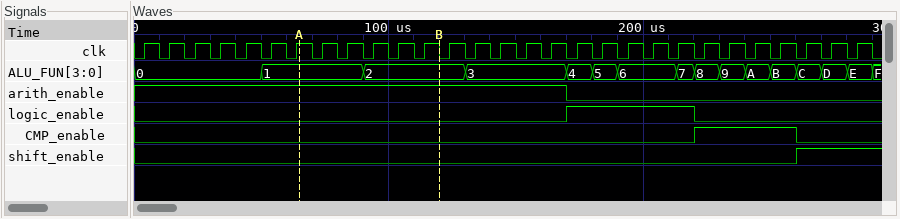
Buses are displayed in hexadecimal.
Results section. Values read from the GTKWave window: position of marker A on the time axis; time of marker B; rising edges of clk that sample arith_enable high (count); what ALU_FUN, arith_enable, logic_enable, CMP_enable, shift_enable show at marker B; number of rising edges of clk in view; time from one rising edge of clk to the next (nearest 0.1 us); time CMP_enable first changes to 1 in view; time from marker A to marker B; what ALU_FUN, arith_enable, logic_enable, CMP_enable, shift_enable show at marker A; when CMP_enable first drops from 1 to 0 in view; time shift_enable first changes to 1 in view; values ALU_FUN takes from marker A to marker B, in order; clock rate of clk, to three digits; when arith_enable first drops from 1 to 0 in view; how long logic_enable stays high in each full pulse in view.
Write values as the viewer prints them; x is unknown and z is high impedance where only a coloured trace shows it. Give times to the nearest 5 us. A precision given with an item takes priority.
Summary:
65 us
120 us
17
ALU_FUN=2, arith_enable=1, logic_enable=0, CMP_enable=0, shift_enable=0
29
10 us
220 us
55 us
ALU_FUN=1, arith_enable=1, logic_enable=0, CMP_enable=0, shift_enable=0
260 us
260 us
1, 2
100 kHz
170 us
50 us
